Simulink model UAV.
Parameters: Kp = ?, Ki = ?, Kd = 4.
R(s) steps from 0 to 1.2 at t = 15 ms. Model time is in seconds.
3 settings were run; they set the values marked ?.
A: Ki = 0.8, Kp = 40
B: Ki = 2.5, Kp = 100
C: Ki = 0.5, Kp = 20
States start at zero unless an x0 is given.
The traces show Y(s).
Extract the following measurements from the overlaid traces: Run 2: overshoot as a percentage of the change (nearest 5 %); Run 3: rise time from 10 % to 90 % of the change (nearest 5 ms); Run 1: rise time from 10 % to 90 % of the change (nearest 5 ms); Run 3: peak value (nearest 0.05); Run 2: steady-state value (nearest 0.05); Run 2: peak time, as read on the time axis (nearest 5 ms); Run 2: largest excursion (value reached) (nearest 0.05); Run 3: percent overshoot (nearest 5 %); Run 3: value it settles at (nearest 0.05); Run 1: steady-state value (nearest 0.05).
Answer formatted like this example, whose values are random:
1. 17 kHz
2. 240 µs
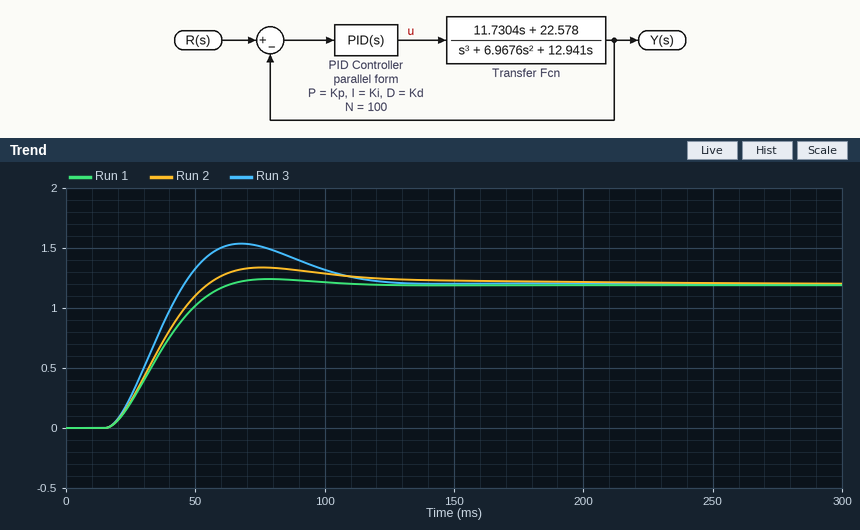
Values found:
1. 10 %
2. 20 ms
3. 30 ms
4. 1.55
5. 1.20
6. 75 ms
7. 1.35
8. 30 %
9. 1.20
10. 1.20
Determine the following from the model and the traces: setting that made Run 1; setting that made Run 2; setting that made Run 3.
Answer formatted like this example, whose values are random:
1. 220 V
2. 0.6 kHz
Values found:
1. C
2. A
3. B
